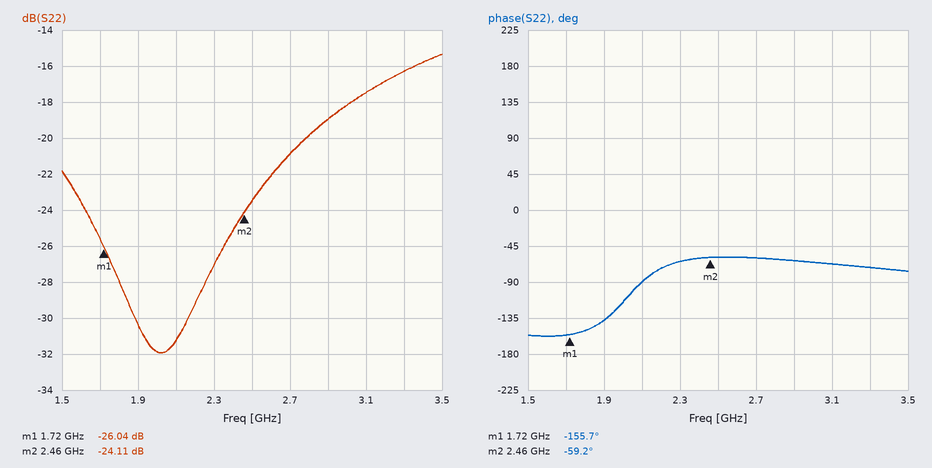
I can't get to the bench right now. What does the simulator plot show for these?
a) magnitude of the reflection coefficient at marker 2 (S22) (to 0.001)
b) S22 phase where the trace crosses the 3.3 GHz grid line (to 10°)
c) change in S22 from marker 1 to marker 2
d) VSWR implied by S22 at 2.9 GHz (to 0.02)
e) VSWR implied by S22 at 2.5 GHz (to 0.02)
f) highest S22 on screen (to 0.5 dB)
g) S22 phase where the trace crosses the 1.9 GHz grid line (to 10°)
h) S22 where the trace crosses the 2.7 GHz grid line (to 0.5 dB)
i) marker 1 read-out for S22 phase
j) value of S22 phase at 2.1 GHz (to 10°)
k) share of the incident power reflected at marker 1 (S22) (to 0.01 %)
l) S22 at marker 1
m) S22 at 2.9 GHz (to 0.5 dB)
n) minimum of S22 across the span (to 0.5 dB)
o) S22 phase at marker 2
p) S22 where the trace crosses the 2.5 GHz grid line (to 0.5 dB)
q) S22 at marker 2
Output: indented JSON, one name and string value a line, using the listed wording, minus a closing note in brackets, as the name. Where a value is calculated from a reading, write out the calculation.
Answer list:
{
  "magnitude of the reflection coefficient at marker 2 (S22)": "10^(-24.11/20) ≈ 0.062",
  "S22 phase where the trace crosses the 3.3 GHz grid line": "-70°",
  "change in S22 from marker 1 to marker 2": "-24.11 − (-26.04) = 1.93 dB",
  "VSWR implied by S22 at 2.9 GHz": "|Γ| = 10^(-19/20) = 0.1122; VSWR = (1 + 0.1122)/(1 − 0.1122) ≈ 1.25, so 1.26 to the nearest 0.02",
  "VSWR implied by S22 at 2.5 GHz": "|Γ| = 10^(-23.5/20) = 0.0668; VSWR = (1 + 0.0668)/(1 − 0.0668) ≈ 1.14",
  "highest S22 on screen": "-15.5 dB",
  "S22 phase where the trace crosses the 1.9 GHz grid line": "-140°",
  "S22 where the trace crosses the 2.7 GHz grid line": "-21.0 dB",
  "marker 1 read-out for S22 phase": "-155.7°",
  "value of S22 phase at 2.1 GHz": "-90°",
  "share of the incident power reflected at marker 1 (S22)": "10^(-26.04/10) ≈ 0.25 %",
  "S22 at marker 1": "-26.04 dB",
  "S22 at 2.9 GHz": "-19.0 dB",
  "minimum of S22 across the span": "-32.0 dB",
  "S22 phase at marker 2": "-59.2°",
  "S22 where the trace crosses the 2.5 GHz grid line": "-23.5 dB",
  "S22 at marker 2": "-24.11 dB"
}
